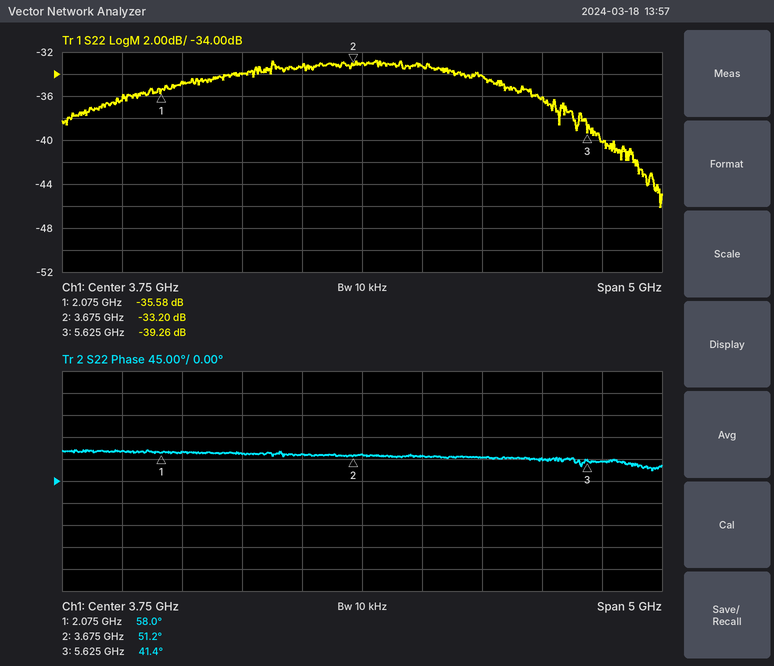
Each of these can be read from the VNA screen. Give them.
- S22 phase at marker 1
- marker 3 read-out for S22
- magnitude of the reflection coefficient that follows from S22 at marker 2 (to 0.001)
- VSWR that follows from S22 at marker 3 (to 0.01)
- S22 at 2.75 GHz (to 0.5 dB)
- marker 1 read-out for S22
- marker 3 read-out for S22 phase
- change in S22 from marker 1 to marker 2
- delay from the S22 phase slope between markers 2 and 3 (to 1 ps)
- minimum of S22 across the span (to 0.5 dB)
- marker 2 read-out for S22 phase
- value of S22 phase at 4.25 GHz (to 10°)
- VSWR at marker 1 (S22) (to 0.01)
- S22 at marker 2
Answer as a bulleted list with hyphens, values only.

- 58.0°
- -39.26 dB
- 0.022
- 1.02
- -34.0 dB
- -35.58 dB
- 41.4°
- 2.38 dB
- 14 ps
- -46.0 dB
- 51.2°
- 50°
- 1.03
- -33.20 dB
